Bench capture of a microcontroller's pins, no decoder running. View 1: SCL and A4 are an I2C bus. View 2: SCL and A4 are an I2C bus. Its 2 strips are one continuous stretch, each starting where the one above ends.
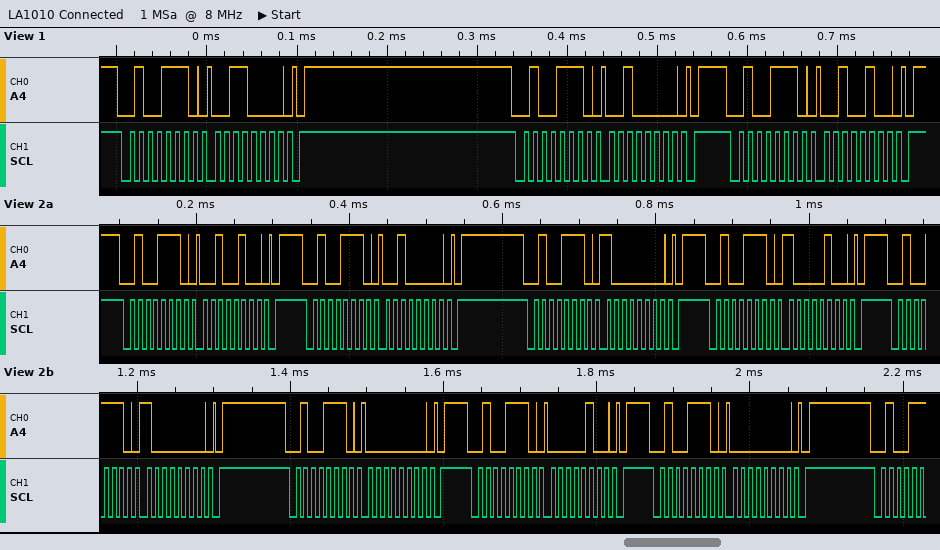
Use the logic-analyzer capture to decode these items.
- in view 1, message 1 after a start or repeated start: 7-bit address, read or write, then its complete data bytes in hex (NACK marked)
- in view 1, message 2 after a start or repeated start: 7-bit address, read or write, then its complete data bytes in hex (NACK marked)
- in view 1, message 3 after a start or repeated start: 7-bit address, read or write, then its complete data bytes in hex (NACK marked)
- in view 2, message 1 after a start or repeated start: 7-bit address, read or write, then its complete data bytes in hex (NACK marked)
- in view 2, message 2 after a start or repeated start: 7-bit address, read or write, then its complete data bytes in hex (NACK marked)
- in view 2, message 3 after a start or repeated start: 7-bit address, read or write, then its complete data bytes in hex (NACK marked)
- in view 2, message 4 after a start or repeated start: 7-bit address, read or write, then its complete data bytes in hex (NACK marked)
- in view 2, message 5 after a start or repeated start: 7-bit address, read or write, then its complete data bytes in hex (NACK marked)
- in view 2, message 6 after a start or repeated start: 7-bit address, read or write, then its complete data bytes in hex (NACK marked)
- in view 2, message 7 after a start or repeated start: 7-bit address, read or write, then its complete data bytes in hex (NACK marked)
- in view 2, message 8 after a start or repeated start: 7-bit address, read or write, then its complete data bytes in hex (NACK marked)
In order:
0x27 write: 30
0x27 write: 20
0x27 write: 24
0x27 write: 24
0x27 write: 20
0x27 write: 80
0x27 write: 84
0x27 write: 80
0x27 write: 00
0x27 write: 04
0x27 write: 00
